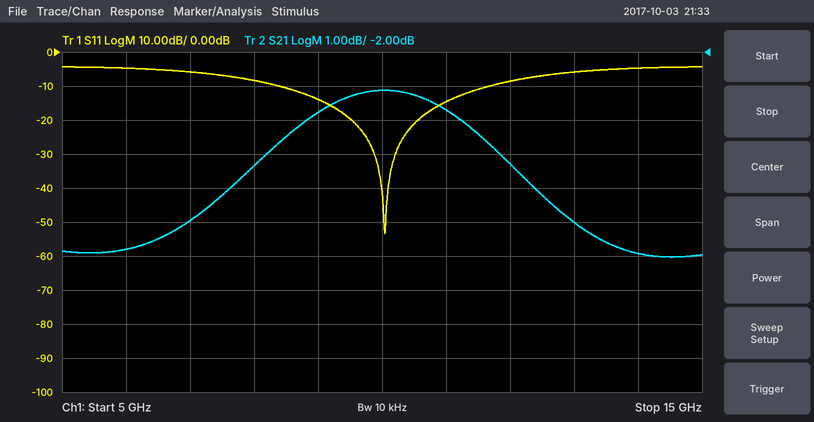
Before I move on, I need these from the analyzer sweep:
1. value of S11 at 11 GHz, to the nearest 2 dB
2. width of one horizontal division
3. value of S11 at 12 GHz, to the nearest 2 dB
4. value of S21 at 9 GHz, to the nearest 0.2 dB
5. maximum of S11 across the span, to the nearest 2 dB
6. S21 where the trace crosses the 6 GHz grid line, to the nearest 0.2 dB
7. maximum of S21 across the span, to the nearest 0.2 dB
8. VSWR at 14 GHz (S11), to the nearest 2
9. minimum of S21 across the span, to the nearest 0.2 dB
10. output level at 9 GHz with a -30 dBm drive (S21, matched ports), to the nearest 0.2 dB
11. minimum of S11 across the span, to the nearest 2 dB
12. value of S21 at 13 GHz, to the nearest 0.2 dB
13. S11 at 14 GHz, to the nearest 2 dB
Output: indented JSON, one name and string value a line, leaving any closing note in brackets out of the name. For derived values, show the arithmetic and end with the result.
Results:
{
  "value of S11 at 11 GHz, to the nearest 2 dB": "-14 dB",
  "width of one horizontal division": "1 GHz",
  "value of S11 at 12 GHz, to the nearest 2 dB": "-8 dB",
  "value of S21 at 9 GHz, to the nearest 0.2 dB": "-3.8 dB",
  "maximum of S11 across the span, to the nearest 2 dB": "-4 dB",
  "S21 where the trace crosses the 6 GHz grid line, to the nearest 0.2 dB": "-7.8 dB",
  "maximum of S21 across the span, to the nearest 0.2 dB": "-3.2 dB",
  "VSWR at 14 GHz (S11), to the nearest 2": "|Γ| = 10^(-4/20) = 0.6310; VSWR = (1 + 0.6310)/(1 − 0.6310) ≈ 4",
  "minimum of S21 across the span, to the nearest 0.2 dB": "-8.0 dB",
  "output level at 9 GHz with a -30 dBm drive (S21, matched ports), to the nearest 0.2 dB": "-30 dBm + (-3.8 dB) = -33.8 dBm",
  "minimum of S11 across the span, to the nearest 2 dB": "-54 dB",
  "value of S21 at 13 GHz, to the nearest 0.2 dB": "-7.0 dB",
  "S11 at 14 GHz, to the nearest 2 dB": "-4 dB"
}
